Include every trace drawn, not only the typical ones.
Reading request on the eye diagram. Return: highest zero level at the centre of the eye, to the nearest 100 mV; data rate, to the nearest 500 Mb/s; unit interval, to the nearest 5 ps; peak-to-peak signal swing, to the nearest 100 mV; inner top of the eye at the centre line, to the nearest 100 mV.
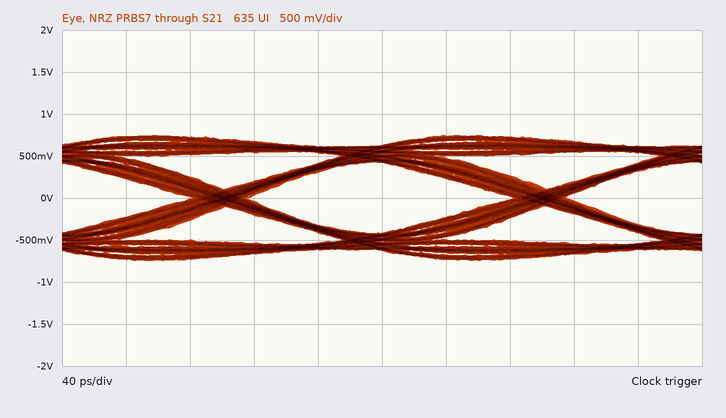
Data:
-400 mV
5.0 Gb/s
200 ps
1.5 V
400 mV
